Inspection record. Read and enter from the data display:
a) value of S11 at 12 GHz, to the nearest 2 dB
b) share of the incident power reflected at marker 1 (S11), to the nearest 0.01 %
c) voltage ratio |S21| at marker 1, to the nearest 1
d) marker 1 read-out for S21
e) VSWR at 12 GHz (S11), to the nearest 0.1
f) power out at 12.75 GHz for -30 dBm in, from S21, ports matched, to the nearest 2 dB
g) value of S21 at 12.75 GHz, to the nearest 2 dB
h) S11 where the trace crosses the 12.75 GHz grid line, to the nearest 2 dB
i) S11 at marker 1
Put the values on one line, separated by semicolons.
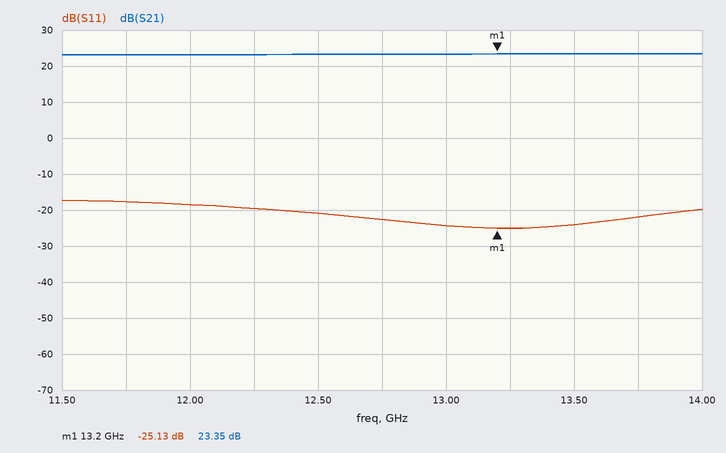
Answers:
-18 dB; 0.31 %; 15; 23.35 dB; 1.3; -6 dBm; 24 dB; -22 dB; -25.13 dB
